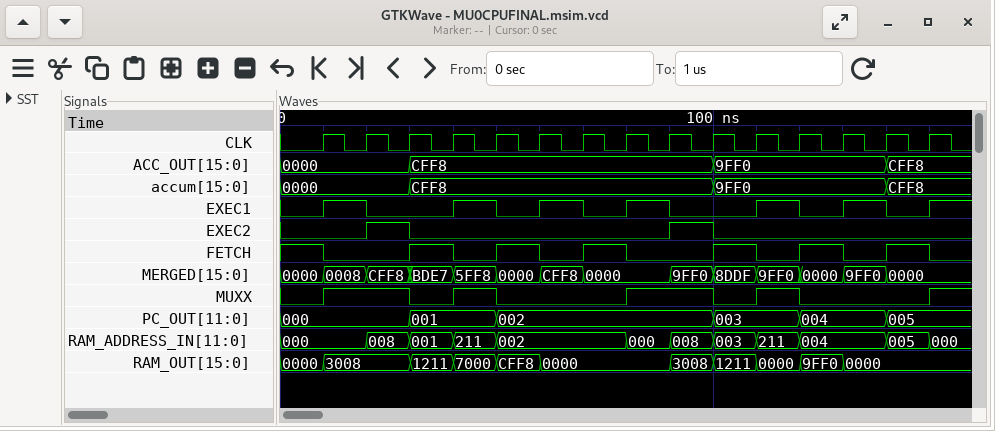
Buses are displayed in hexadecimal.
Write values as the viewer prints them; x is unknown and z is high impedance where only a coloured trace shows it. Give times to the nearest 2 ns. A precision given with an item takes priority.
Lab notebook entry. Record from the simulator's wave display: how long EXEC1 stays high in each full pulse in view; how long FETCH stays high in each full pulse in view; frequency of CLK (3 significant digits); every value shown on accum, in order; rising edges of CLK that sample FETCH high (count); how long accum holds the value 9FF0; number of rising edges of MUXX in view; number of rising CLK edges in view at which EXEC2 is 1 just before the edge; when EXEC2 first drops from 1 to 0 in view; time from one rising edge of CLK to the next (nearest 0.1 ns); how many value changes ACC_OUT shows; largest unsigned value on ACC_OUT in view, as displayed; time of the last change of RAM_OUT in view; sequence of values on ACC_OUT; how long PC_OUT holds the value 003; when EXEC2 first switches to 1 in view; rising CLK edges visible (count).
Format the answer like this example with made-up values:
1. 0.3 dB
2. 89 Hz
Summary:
1. 10 ns, 10 ns, 10 ns, 10 ns, 10 ns, 10 ns
2. 10 ns, 10 ns, 10 ns, 10 ns, 10 ns, 10 ns
3. 100 MHz
4. 0000, CFF8, 9FF0, CFF8
5. 7
6. 40 ns
7. 5
8. 2
9. 30 ns
10. 10 ns
11. 3
12. CFF8
13. 130 ns
14. 0000, CFF8, 9FF0, CFF8
15. 20 ns
16. 20 ns
17. 15
